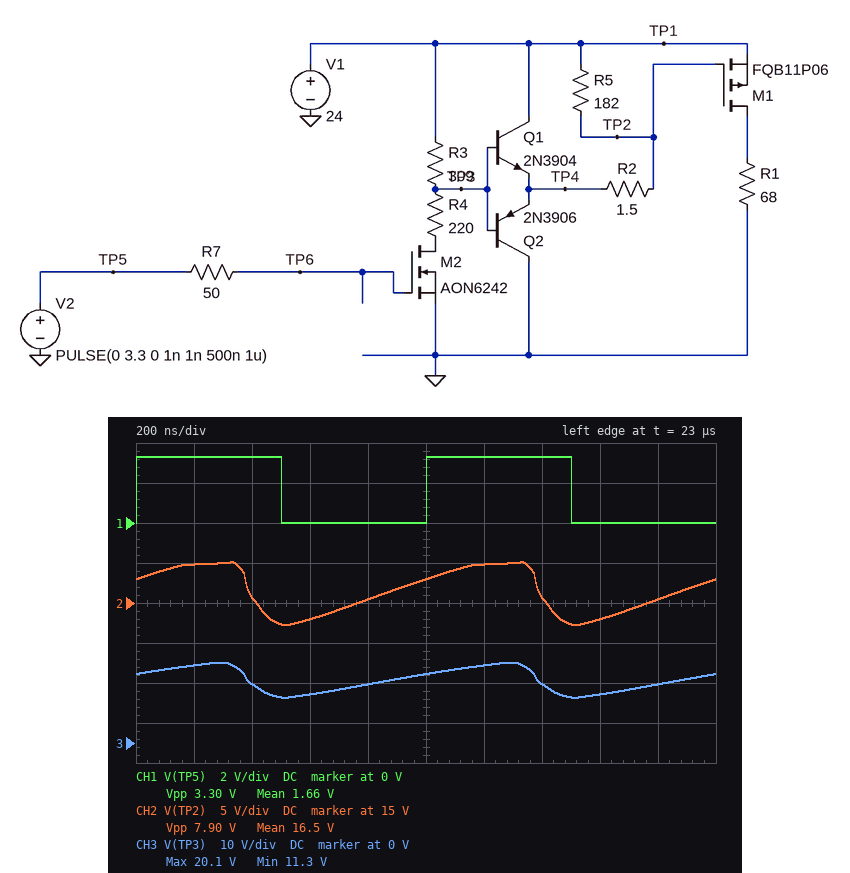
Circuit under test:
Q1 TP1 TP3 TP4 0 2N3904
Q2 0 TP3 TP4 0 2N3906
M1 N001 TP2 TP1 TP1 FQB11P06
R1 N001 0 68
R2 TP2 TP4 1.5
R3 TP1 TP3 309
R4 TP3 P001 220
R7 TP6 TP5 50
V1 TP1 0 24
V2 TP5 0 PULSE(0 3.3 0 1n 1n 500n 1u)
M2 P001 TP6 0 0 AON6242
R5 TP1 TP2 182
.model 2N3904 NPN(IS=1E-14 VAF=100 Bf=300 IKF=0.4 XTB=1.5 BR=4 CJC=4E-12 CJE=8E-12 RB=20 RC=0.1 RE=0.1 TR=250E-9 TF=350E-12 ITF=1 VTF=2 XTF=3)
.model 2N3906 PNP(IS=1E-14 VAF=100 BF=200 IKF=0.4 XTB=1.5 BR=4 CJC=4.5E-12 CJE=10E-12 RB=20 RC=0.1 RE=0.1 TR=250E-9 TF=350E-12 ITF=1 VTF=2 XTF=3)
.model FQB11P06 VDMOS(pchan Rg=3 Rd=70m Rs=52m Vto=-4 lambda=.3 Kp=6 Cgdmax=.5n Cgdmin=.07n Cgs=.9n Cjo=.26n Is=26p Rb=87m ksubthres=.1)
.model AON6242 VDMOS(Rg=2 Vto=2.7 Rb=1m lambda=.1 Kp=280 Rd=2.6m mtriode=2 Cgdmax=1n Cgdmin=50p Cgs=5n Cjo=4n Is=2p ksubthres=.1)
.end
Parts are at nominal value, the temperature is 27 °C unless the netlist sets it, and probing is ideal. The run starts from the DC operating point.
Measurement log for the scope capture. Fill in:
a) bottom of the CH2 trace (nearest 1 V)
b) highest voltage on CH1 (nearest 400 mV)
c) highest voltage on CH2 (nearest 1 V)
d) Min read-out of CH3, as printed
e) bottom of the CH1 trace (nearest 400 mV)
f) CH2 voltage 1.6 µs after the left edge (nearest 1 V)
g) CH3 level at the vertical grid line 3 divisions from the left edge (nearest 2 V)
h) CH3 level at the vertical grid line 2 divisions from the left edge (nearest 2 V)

12 V
3.2 V
20 V
11.3 V
0 V
13 V
12 V
14 V
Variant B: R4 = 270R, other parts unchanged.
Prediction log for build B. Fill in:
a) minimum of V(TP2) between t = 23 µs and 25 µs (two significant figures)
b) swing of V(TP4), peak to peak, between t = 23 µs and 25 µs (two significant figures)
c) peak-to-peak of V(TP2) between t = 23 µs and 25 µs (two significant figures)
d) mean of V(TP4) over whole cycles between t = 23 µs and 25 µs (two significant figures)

13 V
6.9 V
6.8 V
17 V
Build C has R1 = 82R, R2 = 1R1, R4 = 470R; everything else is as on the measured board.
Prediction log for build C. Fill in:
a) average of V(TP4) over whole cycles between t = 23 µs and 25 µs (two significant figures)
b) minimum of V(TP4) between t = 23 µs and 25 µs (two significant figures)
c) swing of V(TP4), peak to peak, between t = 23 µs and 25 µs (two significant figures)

18 V
16 V
4.0 V
